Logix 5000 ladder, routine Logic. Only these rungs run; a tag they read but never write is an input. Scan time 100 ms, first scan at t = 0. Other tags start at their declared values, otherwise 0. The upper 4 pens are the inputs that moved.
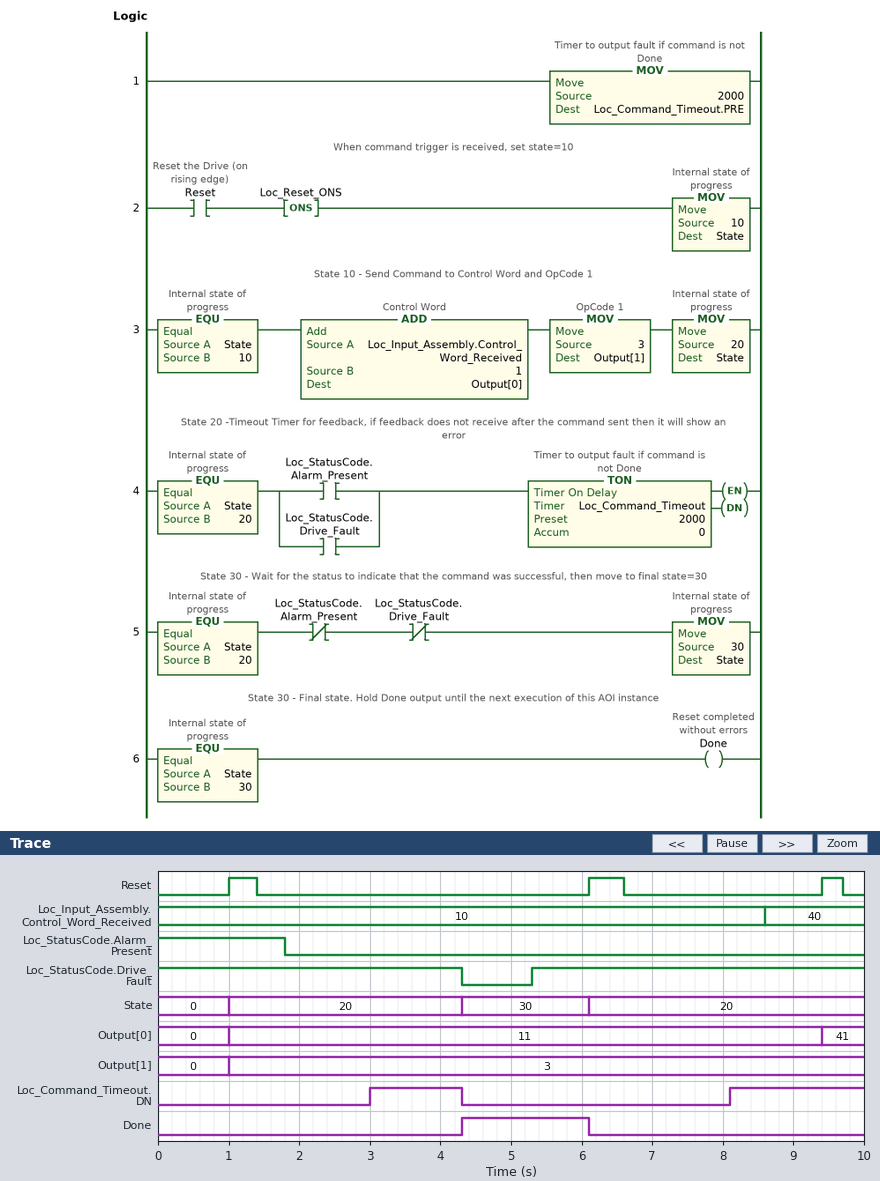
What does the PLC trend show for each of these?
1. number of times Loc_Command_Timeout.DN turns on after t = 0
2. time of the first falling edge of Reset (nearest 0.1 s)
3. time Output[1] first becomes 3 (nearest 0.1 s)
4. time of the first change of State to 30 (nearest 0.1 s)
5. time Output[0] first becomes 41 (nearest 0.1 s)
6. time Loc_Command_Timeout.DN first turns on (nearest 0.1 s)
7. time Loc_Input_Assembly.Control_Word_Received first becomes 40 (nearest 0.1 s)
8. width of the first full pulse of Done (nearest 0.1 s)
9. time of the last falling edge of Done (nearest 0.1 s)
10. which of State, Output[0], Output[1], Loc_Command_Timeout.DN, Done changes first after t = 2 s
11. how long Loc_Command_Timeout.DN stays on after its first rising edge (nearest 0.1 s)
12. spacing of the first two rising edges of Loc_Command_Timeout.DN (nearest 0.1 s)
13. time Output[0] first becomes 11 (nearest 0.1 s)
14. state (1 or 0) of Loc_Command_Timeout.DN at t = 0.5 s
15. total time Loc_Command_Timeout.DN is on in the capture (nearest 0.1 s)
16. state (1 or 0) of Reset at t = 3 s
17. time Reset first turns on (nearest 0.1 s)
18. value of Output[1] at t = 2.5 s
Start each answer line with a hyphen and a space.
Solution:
- 2
- 1.4 s
- 1.0 s
- 4.3 s
- 9.4 s
- 3.0 s
- 8.6 s
- 1.8 s
- 6.1 s
- Loc_Command_Timeout.DN
- 1.3 s
- 5.1 s
- 1.0 s
- 0
- 3.2 s
- 0
- 1.0 s
- 3
